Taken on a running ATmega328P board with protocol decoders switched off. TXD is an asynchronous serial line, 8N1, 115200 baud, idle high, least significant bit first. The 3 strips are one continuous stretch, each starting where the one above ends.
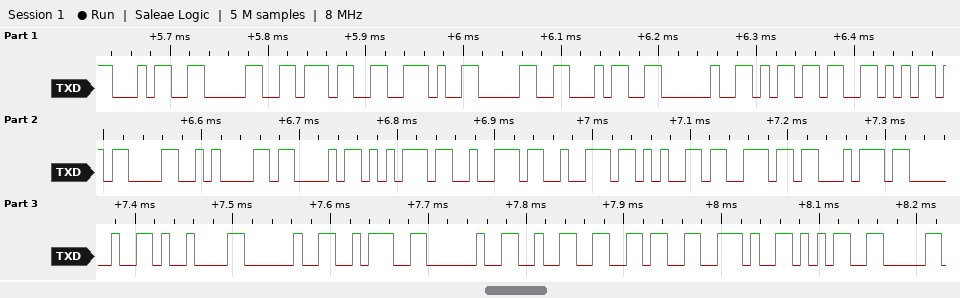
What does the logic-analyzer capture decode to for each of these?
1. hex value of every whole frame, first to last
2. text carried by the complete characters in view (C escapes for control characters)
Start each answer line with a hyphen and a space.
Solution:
- 34 30 37 2E 30 34 20 6D 56 0D 0A 43 75 72 72 65 6E 74 20 09 20 3A 20 32 36 2E 35
- "407.04 mV\r\nCurrent \t : 26.5"
